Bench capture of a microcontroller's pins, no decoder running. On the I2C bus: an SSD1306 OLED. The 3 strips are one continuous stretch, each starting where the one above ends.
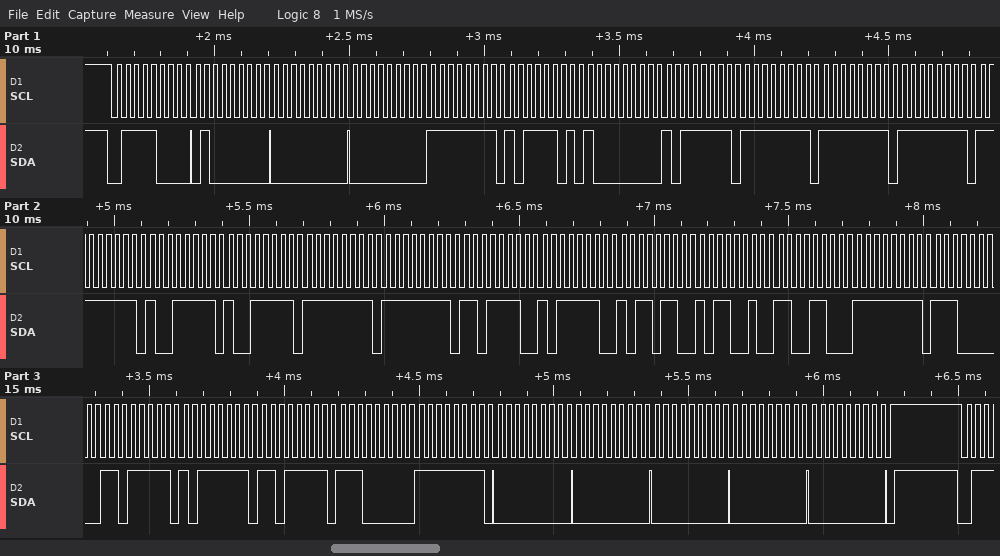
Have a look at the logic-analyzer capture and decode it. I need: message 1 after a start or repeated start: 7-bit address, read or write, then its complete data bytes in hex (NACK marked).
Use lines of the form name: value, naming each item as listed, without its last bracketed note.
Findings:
message 1 after a start or repeated start: 7-bit address, read or write, then its complete data bytes in hex: 0x3C write: 40 00 00 FF BD 80 BF FF FF FF FF 9F 9F FF FF DE BE B6 B2 CC FF E0 DF BF DF E0 FF 00 00 00 00 00
